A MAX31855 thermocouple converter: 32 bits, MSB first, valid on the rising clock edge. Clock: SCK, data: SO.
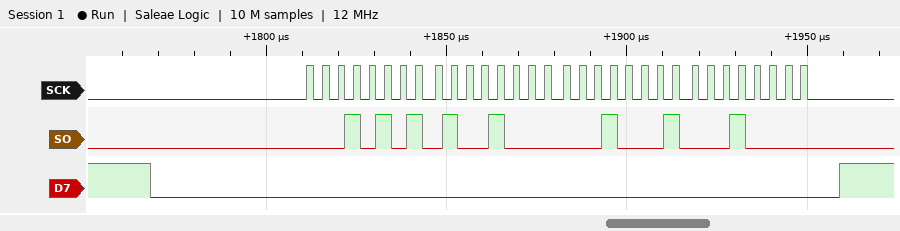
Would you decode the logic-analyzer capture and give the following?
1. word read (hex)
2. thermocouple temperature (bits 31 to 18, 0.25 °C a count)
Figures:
0x15481110
340.50 °C
